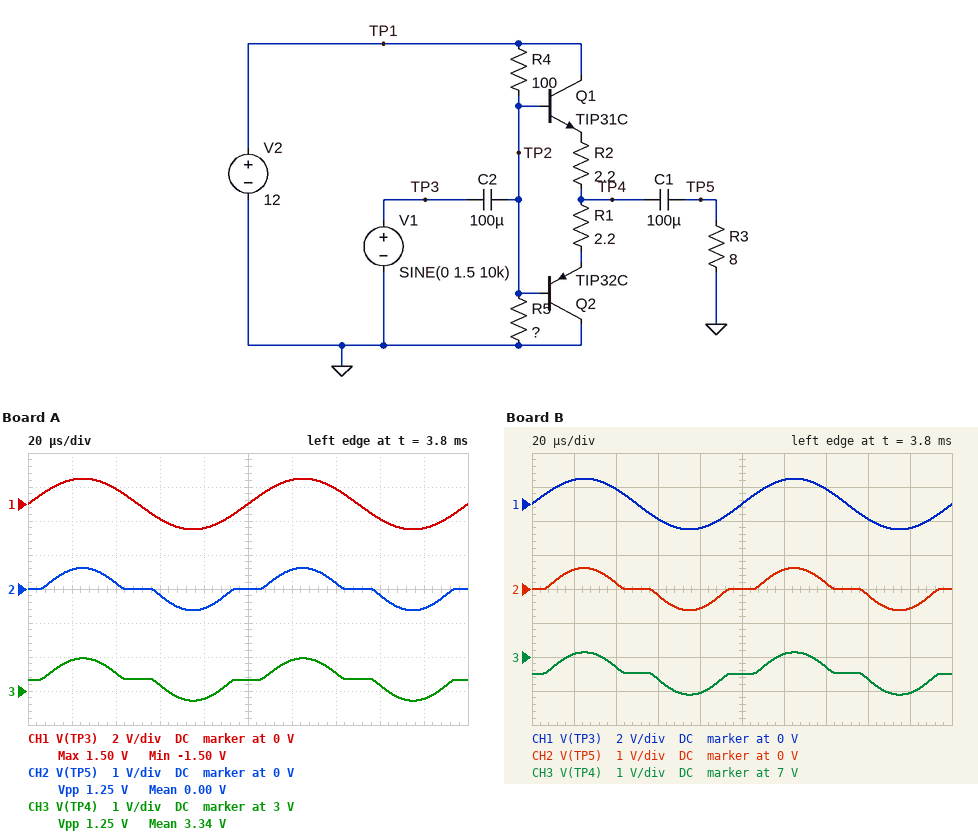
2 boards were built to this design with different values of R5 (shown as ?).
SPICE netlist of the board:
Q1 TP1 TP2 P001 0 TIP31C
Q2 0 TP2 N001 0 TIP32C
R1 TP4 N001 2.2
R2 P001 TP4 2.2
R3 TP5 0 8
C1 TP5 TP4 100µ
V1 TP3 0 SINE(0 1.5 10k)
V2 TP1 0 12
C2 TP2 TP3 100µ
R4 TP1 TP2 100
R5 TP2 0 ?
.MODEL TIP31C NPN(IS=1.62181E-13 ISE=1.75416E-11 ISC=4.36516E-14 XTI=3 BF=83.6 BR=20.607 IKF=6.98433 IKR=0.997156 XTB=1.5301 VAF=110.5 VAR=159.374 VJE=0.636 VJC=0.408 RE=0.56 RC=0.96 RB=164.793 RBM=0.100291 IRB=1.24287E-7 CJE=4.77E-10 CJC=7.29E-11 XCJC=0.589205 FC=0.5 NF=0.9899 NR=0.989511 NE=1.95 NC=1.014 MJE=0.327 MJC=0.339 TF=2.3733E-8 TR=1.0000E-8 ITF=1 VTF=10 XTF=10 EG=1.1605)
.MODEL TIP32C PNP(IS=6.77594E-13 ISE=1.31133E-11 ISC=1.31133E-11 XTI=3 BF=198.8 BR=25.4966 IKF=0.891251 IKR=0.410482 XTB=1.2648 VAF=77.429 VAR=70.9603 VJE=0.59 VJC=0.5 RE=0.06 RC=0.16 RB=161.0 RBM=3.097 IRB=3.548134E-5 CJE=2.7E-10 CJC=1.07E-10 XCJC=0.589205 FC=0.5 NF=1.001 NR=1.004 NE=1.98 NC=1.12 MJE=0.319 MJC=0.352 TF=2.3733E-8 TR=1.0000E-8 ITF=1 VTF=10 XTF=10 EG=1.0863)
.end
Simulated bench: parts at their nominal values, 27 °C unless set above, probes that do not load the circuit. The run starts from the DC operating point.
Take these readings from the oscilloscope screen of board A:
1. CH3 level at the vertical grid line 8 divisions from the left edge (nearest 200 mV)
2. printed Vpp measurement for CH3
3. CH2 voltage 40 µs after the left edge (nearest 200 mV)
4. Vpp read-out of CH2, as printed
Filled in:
3.2 V
1.25 V
200 mV
1.25 V
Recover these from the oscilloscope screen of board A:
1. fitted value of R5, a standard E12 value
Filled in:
39 Ω
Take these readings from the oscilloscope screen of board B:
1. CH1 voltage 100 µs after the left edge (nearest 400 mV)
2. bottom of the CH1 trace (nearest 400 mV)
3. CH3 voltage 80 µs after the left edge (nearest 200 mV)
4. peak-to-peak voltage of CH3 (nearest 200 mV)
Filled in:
0 V
-1.6 V
6.0 V
1.2 V
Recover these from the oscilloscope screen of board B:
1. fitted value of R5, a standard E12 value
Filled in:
120 Ω
